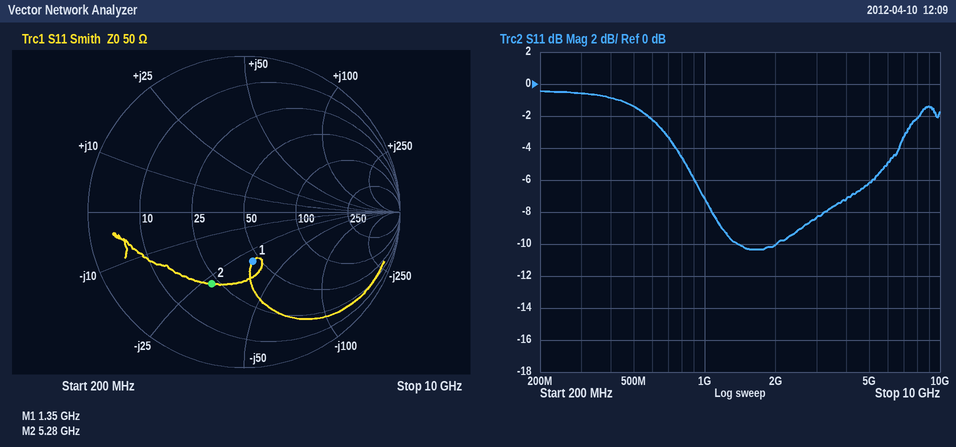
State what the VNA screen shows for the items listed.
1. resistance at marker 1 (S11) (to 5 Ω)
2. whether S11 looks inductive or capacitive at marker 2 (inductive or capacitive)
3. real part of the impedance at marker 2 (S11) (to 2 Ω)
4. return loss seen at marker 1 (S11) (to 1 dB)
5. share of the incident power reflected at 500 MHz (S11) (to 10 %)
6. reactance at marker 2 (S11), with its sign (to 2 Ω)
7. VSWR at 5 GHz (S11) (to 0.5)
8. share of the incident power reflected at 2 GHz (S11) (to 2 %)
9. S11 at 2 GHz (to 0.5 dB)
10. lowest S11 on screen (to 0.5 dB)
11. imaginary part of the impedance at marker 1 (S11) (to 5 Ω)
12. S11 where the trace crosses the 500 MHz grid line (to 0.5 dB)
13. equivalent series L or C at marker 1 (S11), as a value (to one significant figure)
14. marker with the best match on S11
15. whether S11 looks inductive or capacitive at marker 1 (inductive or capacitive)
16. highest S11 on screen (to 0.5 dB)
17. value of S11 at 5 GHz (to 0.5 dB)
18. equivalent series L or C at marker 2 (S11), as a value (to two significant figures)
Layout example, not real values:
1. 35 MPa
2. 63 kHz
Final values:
1. 45 Ω
2. capacitive
3. 22 Ω
4. 10 dB
5. 70 %
6. -28 Ω
7. 3.0
8. 10 %
9. -10.0 dB
10. -10.5 dB
11. -30 Ω
12. -1.5 dB
13. 4 pF
14. marker 1
15. capacitive
16. -0.5 dB
17. -6.0 dB
18. 1.1 pF
